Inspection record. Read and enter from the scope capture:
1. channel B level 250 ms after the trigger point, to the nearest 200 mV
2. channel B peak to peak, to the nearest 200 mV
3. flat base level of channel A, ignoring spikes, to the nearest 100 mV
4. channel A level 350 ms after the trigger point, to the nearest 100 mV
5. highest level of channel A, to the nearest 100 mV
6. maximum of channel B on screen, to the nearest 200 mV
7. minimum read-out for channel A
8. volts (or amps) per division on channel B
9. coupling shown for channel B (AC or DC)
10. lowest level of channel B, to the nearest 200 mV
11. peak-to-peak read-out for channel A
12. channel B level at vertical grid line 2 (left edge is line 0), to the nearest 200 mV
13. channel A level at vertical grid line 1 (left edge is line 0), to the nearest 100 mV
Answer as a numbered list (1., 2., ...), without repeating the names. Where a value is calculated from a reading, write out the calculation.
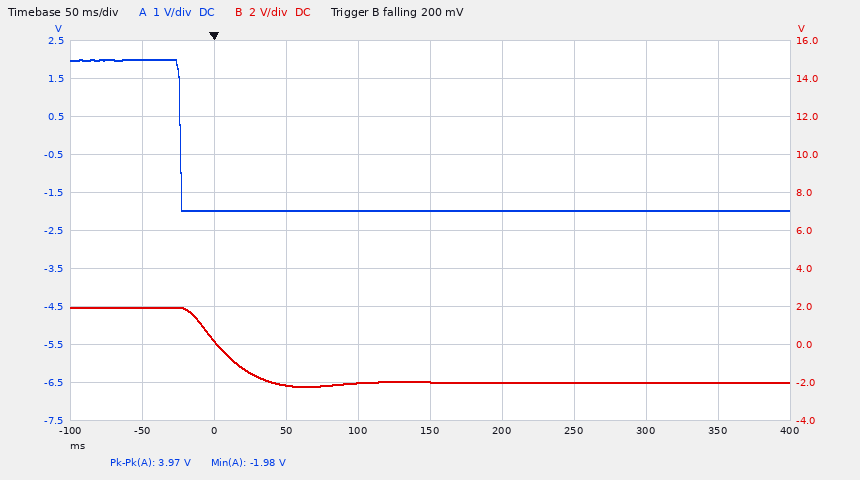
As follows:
1. -2.0 V
2. 2.0 V − (-2.2 V) = 4.2 V
3. -2.0 V
4. -2.0 V
5. 2.0 V
6. 2.0 V
7. -1.98 V
8. 2 V
9. DC
10. -2.2 V
11. 3.97 V
12. 200 mV
13. 2.0 V
